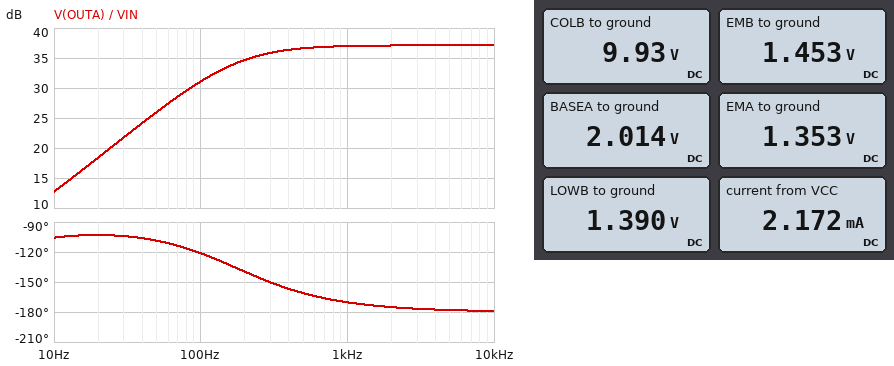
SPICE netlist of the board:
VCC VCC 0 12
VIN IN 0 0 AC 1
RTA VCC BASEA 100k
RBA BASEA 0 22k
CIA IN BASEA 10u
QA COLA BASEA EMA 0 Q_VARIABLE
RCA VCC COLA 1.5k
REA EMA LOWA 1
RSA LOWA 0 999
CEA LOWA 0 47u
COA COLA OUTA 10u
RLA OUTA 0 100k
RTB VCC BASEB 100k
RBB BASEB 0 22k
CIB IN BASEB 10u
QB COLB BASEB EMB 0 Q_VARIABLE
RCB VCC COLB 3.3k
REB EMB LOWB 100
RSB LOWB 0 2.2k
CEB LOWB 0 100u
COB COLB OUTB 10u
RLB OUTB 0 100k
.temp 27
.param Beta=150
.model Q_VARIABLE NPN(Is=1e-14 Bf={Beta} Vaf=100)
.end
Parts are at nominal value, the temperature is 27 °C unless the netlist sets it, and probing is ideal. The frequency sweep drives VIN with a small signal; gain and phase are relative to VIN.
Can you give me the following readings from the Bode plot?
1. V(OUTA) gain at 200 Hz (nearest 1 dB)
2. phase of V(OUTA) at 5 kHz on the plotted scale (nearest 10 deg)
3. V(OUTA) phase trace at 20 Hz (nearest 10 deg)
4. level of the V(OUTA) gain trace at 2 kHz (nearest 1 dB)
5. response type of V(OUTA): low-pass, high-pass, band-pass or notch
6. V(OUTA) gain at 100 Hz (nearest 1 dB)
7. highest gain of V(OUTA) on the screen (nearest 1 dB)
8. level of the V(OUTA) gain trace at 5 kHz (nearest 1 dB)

35 dB
-180 deg
-100 deg
37 dB
high-pass
31 dB
37 dB
37 dB
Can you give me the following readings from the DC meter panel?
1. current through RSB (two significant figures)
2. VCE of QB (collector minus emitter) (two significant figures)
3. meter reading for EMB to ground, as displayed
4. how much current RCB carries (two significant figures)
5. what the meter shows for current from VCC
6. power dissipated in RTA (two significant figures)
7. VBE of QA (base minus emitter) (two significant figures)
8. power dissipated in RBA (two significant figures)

630 µA
8.5 V
1.453 V
630 µA
2.172 mA
1.0 mW
660 mV
180 µW
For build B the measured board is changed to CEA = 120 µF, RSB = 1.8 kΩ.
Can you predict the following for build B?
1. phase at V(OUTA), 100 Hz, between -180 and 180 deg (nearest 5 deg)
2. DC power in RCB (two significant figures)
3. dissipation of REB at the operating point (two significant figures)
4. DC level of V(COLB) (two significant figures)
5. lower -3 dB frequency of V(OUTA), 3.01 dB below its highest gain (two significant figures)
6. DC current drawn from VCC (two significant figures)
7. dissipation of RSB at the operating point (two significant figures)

-145 deg
1.9 mW
57 µW
9.5 V
71 Hz
2.3 mA
1.0 mW
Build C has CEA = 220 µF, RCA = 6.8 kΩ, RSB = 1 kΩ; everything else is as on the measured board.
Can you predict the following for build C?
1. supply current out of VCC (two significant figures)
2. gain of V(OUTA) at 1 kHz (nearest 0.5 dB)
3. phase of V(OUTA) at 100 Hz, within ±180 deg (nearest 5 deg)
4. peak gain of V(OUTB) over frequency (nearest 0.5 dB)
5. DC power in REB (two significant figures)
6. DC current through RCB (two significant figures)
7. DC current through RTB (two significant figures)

2.8 mA
49.0 dB
-160 deg
28.5 dB
150 µW
1.2 mA
100 µA
